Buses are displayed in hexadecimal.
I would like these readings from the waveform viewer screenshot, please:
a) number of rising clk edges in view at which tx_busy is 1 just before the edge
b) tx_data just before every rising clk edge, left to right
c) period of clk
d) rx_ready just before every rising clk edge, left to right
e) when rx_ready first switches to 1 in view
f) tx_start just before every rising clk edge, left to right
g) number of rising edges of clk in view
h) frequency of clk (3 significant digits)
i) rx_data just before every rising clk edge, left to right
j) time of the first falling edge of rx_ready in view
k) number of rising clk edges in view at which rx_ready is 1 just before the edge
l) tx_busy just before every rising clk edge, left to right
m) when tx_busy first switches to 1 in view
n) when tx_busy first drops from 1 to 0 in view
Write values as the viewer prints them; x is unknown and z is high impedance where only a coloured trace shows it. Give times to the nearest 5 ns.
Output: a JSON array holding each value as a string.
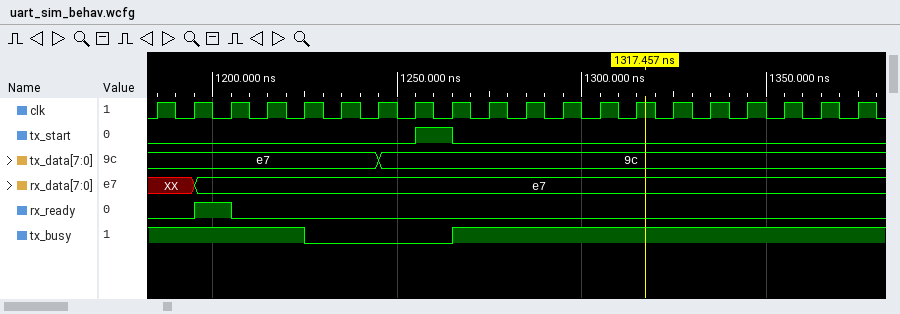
["16", "e7, e7, e7, e7, e7, e7, e7, 9c, 9c, 9c, 9c, 9c, 9c, 9c, 9c, 9c, 9c, 9c, 9c, 9c", "10 ns", "0 0 1 0 0 0 0 0 0 0 0 0 0 0 0 0 0 0 0 0", "1195 ns", "0 0 0 0 0 0 0 0 1 0 0 0 0 0 0 0 0 0 0 0", "20", "100 MHz", "XX, XX, e7, e7, e7, e7, e7, e7, e7, e7, e7, e7, e7, e7, e7, e7, e7, e7, e7, e7", "1205 ns", "1", "1 1 1 1 1 0 0 0 0 1 1 1 1 1 1 1 1 1 1 1", "1265 ns", "1225 ns"]
